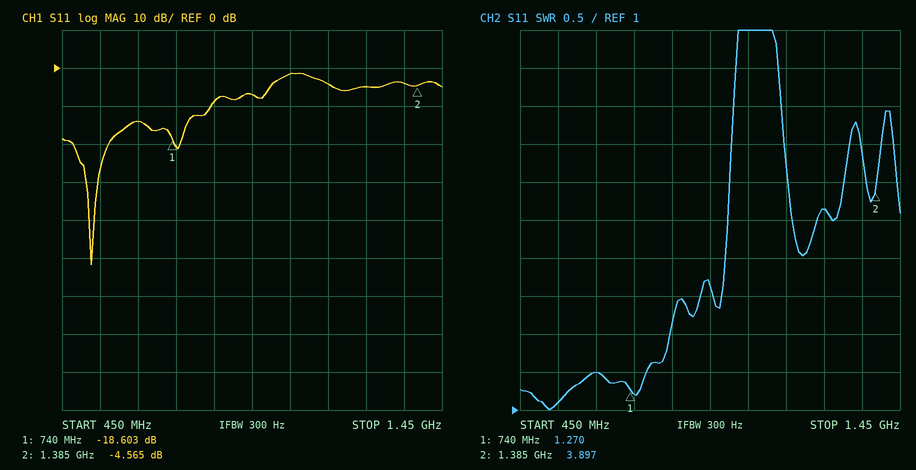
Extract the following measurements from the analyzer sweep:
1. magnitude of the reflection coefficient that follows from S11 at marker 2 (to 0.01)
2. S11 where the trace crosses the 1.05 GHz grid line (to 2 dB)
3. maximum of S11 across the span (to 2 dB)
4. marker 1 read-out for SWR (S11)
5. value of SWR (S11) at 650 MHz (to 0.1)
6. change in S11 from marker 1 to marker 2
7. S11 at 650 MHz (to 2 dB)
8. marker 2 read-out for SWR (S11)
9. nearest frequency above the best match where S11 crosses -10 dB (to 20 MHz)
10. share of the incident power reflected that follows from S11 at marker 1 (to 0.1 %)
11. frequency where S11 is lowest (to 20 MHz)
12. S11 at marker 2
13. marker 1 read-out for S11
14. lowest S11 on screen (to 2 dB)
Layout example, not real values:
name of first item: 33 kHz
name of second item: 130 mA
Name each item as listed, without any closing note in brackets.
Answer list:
magnitude of the reflection coefficient that follows from S11 at marker 2: 0.59
S11 where the trace crosses the 1.05 GHz grid line: -2 dB
maximum of S11 across the span: -2 dB
marker 1 read-out for SWR: 1.270
value of SWR (S11) at 650 MHz: 1.5
change in S11 from marker 1 to marker 2: 14.038 dB
S11 at 650 MHz: -14 dB
marker 2 read-out for SWR: 3.897
nearest frequency above the best match where S11 crosses -10 dB: 840 MHz
share of the incident power reflected that follows from S11 at marker 1: 1.4 %
frequency where S11 is lowest: 520 MHz
S11 at marker 2: -4.565 dB
marker 1 read-out for S11: -18.603 dB
lowest S11 on screen: -52 dB
